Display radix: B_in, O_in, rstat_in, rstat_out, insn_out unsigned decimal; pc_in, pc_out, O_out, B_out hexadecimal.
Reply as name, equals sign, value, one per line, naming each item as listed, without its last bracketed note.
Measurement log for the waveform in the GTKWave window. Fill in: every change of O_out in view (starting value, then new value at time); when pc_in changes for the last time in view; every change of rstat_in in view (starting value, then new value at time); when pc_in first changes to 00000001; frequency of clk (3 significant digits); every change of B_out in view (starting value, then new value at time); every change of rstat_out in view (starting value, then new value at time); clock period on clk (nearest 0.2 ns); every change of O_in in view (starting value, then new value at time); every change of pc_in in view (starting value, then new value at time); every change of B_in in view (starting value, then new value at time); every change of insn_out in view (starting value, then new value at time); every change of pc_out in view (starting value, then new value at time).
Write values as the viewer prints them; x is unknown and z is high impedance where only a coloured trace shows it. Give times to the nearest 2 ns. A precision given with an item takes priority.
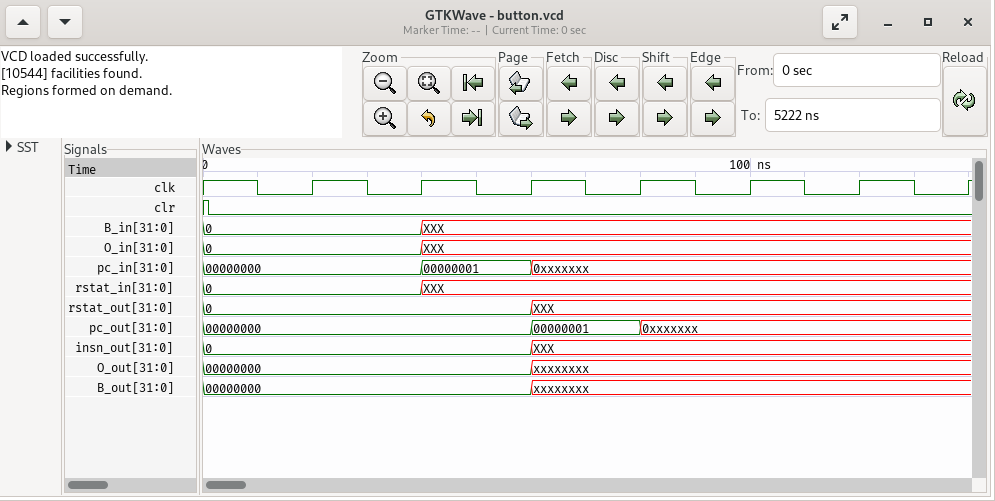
every change of O_out in view = 00000000, xxxxxxxx at 60 ns
when pc_in changes for the last time in view = 60 ns
every change of rstat_in in view = 0, XXX at 40 ns
when pc_in first changes to 00000001 = 40 ns
frequency of clk = 50.0 MHz
every change of B_out in view = 00000000, xxxxxxxx at 60 ns
every change of rstat_out in view = 0, XXX at 60 ns
clock period on clk = 20 ns
every change of O_in in view = 0, XXX at 40 ns
every change of pc_in in view = 00000000, 00000001 at 40 ns, 0xxxxxxx at 60 ns
every change of B_in in view = 0, XXX at 40 ns
every change of insn_out in view = 0, XXX at 60 ns
every change of pc_out in view = 00000000, 00000001 at 60 ns, 0xxxxxxx at 80 ns
